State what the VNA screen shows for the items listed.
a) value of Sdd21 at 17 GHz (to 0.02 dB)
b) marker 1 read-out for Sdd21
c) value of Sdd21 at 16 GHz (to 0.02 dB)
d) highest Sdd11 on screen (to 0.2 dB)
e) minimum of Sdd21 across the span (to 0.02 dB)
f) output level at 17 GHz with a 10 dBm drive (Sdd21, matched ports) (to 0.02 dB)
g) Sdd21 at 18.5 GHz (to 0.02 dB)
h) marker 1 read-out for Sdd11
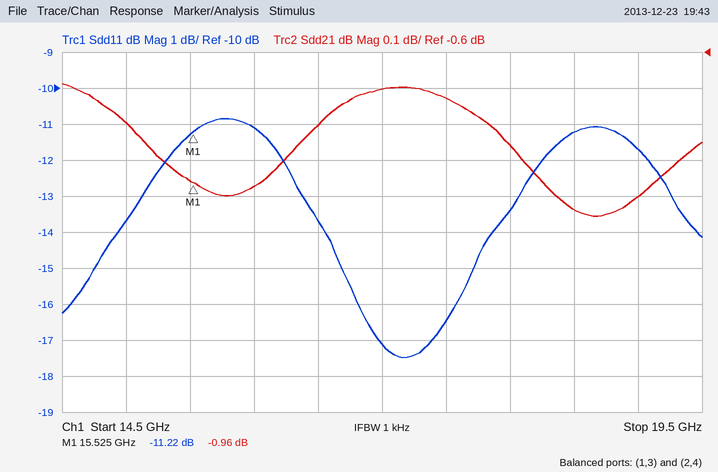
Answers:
-0.70 dB
-0.96 dB
-0.98 dB
-10.8 dB
-1.06 dB
9.30 dBm
-1.04 dB
-11.22 dB
